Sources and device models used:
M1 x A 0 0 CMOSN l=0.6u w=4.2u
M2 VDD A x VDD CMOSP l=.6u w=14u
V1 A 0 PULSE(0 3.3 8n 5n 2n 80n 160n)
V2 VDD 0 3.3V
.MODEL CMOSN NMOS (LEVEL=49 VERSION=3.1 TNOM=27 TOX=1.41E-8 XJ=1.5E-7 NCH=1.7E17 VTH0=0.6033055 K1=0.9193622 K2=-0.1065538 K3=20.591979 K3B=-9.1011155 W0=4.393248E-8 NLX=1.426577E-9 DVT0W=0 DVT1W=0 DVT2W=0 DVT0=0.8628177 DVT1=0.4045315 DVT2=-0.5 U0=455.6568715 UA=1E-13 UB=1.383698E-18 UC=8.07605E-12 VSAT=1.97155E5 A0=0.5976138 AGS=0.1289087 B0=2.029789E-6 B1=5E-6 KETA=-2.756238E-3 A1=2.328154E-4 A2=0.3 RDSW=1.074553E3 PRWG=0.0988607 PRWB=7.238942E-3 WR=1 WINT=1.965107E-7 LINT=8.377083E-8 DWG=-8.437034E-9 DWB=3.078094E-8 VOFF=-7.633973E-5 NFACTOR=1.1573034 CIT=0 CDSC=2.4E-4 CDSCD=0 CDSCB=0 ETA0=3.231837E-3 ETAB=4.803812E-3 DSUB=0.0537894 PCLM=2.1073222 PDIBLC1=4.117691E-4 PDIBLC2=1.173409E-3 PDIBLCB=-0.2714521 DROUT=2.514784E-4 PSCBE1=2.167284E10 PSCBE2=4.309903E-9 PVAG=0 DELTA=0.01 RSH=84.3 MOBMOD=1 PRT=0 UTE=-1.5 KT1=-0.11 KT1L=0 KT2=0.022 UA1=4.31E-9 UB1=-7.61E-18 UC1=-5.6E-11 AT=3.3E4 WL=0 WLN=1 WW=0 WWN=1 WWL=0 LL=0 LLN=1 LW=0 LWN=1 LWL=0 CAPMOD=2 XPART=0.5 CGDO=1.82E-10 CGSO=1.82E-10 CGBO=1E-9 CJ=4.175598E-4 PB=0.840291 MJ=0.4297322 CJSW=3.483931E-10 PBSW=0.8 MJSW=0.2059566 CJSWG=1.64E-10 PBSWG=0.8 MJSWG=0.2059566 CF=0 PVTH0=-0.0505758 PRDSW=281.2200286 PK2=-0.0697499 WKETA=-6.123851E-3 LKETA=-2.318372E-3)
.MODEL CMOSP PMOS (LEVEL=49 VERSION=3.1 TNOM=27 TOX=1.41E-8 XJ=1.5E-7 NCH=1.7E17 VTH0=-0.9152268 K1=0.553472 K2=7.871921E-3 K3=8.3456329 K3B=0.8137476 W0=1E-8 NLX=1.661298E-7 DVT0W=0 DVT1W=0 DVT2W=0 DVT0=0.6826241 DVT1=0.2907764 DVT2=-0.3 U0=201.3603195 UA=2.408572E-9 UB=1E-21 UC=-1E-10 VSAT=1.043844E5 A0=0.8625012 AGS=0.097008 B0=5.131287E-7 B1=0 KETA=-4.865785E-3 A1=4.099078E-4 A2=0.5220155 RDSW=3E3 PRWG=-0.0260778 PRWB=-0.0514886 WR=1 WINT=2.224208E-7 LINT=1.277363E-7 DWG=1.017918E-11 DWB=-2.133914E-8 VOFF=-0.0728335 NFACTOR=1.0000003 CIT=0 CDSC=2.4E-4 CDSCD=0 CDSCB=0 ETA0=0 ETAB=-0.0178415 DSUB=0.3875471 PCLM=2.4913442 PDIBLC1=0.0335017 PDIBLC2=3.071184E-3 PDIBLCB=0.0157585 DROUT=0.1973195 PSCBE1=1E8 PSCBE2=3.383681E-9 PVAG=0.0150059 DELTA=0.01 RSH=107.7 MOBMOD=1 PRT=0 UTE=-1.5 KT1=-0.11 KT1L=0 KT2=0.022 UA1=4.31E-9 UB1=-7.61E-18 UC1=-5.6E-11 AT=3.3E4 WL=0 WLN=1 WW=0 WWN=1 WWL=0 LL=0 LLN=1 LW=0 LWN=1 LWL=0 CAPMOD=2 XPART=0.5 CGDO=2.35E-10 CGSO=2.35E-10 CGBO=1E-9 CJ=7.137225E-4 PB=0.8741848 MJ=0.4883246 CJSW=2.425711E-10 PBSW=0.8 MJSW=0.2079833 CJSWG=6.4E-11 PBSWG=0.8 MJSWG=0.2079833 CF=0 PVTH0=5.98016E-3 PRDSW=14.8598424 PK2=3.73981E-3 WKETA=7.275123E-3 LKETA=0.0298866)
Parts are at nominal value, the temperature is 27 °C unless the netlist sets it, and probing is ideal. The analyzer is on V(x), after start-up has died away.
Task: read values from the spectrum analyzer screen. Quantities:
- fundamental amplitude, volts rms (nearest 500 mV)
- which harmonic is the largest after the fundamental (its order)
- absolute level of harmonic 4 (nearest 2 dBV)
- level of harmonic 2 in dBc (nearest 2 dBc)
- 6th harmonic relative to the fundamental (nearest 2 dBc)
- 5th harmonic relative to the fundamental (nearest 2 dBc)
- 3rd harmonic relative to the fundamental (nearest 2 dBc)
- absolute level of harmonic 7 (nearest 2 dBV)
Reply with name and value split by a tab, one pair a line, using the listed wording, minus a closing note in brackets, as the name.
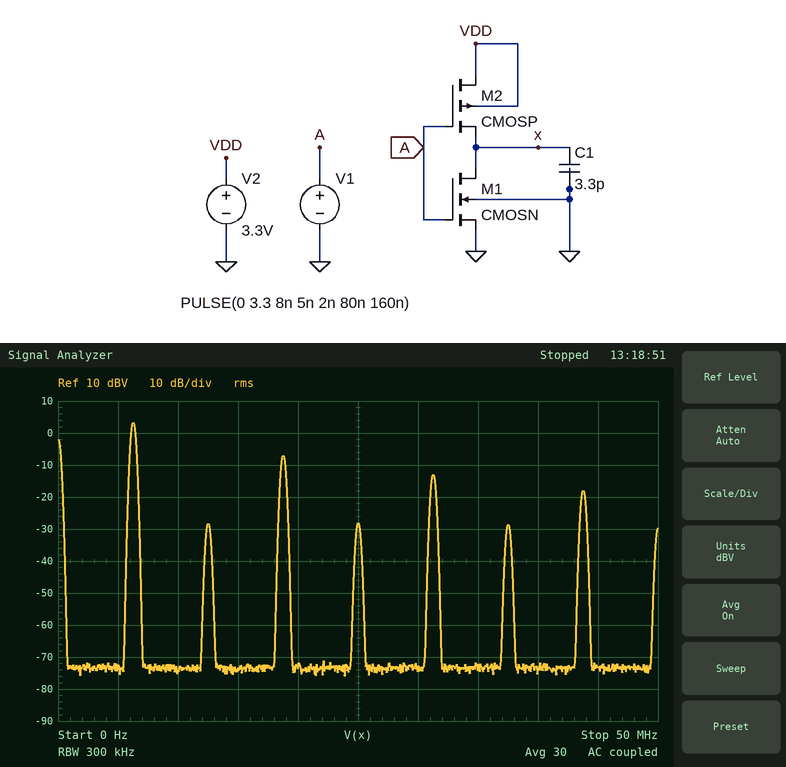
fundamental amplitude, volts rms	1.5 V
which harmonic is the largest after the fundamental	3
absolute level of harmonic 4	-28 dBV
level of harmonic 2 in dBc	-32 dBc
6th harmonic relative to the fundamental	-32 dBc
5th harmonic relative to the fundamental	-16 dBc
3rd harmonic relative to the fundamental	-10 dBc
absolute level of harmonic 7	-18 dBV
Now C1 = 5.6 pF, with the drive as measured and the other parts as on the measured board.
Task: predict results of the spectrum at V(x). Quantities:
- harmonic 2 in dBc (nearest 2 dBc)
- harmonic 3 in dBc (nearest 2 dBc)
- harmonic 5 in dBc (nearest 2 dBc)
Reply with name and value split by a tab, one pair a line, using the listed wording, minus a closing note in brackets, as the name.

harmonic 2 in dBc	-36 dBc
harmonic 3 in dBc	-12 dBc
harmonic 5 in dBc	-20 dBc
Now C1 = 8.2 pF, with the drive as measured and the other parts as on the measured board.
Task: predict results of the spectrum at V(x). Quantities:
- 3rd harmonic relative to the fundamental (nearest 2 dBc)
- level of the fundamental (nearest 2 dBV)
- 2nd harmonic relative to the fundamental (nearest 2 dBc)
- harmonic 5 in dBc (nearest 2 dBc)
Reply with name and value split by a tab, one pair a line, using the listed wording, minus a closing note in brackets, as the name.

3rd harmonic relative to the fundamental	-14 dBc
level of the fundamental	2 dBV
2nd harmonic relative to the fundamental	-30 dBc
harmonic 5 in dBc	-24 dBc
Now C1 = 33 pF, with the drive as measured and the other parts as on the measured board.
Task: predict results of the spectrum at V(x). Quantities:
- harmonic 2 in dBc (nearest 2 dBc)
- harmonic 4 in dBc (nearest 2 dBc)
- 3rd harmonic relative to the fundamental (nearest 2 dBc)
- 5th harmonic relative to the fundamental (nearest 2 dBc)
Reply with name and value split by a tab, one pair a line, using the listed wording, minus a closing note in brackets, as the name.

harmonic 2 in dBc	-22 dBc
harmonic 4 in dBc	-34 dBc
3rd harmonic relative to the fundamental	-20 dBc
5th harmonic relative to the fundamental	-30 dBc
